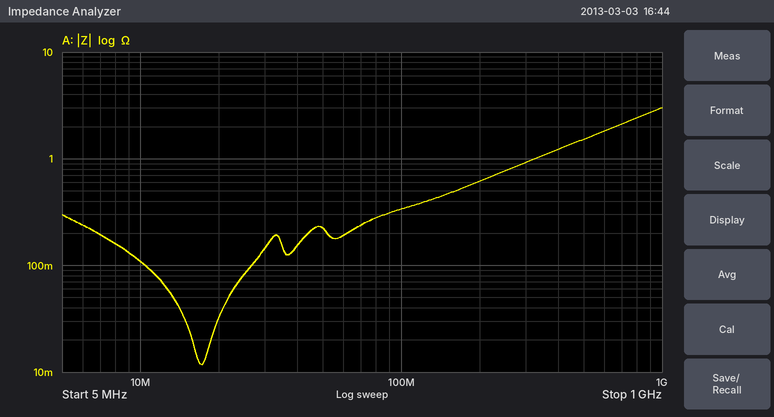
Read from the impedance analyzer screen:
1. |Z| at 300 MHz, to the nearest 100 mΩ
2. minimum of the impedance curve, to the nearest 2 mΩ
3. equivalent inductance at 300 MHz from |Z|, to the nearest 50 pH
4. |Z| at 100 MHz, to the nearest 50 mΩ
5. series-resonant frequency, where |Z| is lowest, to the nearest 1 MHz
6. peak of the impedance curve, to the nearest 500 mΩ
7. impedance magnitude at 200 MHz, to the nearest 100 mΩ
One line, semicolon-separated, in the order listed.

900 mΩ; 12 mΩ; 500 pH; 350 mΩ; 17 MHz; 3.0 Ω; 600 mΩ
